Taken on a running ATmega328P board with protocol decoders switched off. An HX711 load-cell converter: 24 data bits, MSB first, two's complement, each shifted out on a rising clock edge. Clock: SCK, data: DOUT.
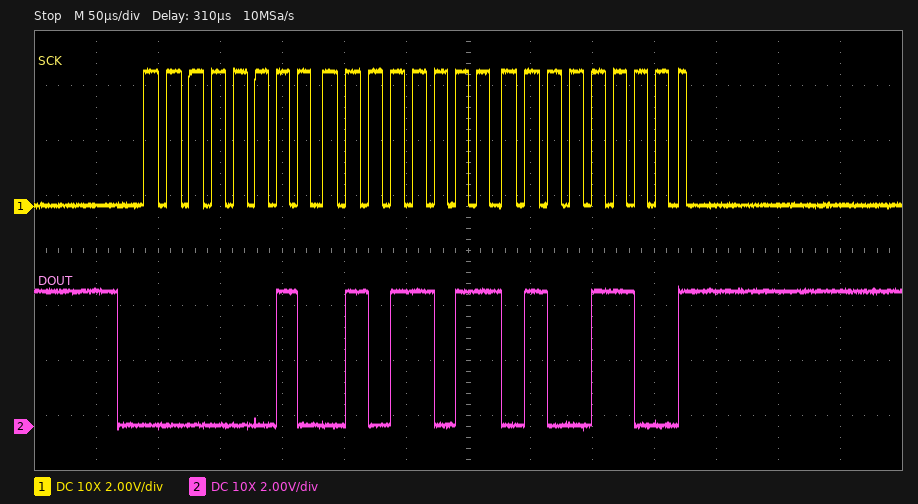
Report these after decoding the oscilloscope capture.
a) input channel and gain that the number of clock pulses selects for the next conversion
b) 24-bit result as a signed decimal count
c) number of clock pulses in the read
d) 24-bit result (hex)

channel A, gain 128
154444
25
0x025B4C
